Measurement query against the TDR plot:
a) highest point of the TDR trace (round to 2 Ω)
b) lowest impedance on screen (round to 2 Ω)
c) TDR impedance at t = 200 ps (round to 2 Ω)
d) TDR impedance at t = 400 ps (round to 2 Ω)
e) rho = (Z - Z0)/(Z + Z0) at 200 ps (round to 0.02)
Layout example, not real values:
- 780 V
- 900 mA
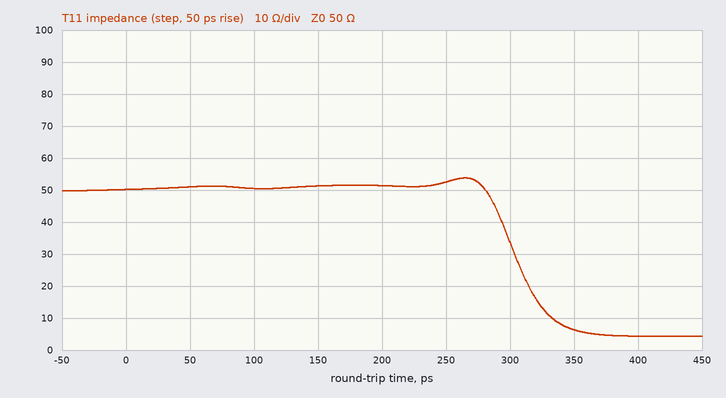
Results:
- 54 Ω
- 4 Ω
- 52 Ω
- 4 Ω
- +0.02
